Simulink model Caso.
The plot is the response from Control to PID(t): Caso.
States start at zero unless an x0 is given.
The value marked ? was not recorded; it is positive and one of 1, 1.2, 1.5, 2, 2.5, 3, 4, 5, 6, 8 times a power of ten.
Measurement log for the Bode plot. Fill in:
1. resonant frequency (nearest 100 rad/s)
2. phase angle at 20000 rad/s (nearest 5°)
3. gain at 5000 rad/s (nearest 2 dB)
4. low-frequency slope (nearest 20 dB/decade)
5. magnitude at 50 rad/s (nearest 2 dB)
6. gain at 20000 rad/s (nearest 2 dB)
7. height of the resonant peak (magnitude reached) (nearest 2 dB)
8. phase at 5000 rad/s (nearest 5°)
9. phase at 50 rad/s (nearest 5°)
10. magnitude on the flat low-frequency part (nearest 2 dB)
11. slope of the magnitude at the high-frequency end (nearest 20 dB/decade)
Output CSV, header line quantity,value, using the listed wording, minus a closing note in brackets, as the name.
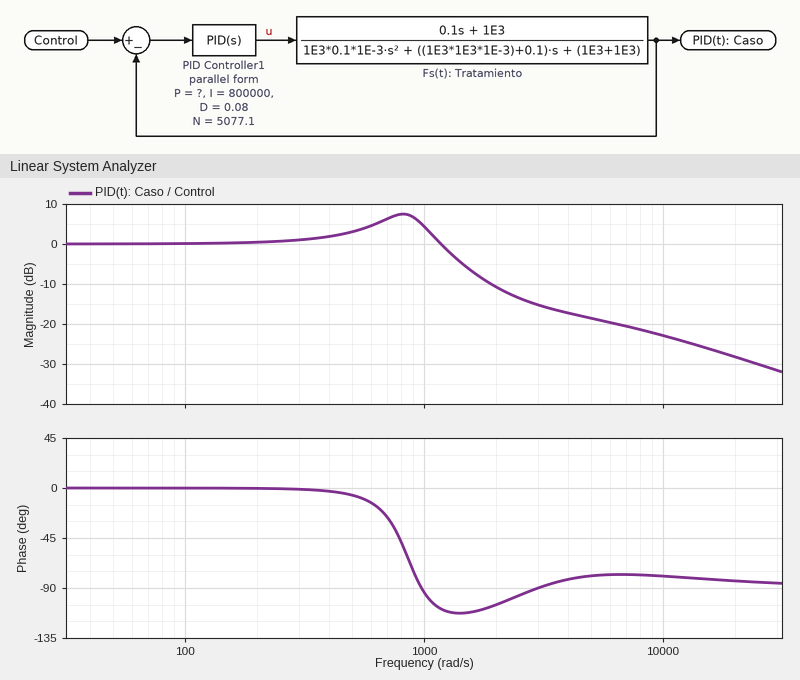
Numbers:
quantity,value
resonant frequency,800 rad/s
phase angle at 20000 rad/s,-85°
gain at 5000 rad/s,-18 dB
low-frequency slope,0 dB/decade
magnitude at 50 rad/s,0 dB
gain at 20000 rad/s,-28 dB
height of the resonant peak (magnitude reached),8 dB
phase at 5000 rad/s,-80°
phase at 50 rad/s,0°
magnitude on the flat low-frequency part,0 dB
slope of the magnitude at the high-frequency end,-20 dB/decade
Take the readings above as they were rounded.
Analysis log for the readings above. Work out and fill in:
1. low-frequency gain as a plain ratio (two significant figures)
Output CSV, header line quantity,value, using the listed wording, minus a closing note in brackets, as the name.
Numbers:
quantity,value
low-frequency gain as a plain ratio,1.0
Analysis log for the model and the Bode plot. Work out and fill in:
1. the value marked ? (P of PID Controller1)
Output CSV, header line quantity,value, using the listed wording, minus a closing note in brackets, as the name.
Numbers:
quantity,value
the value marked ?,400
